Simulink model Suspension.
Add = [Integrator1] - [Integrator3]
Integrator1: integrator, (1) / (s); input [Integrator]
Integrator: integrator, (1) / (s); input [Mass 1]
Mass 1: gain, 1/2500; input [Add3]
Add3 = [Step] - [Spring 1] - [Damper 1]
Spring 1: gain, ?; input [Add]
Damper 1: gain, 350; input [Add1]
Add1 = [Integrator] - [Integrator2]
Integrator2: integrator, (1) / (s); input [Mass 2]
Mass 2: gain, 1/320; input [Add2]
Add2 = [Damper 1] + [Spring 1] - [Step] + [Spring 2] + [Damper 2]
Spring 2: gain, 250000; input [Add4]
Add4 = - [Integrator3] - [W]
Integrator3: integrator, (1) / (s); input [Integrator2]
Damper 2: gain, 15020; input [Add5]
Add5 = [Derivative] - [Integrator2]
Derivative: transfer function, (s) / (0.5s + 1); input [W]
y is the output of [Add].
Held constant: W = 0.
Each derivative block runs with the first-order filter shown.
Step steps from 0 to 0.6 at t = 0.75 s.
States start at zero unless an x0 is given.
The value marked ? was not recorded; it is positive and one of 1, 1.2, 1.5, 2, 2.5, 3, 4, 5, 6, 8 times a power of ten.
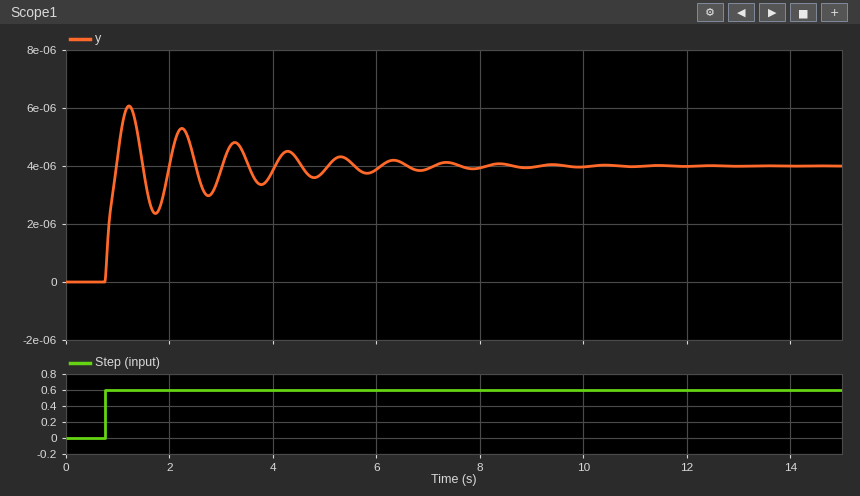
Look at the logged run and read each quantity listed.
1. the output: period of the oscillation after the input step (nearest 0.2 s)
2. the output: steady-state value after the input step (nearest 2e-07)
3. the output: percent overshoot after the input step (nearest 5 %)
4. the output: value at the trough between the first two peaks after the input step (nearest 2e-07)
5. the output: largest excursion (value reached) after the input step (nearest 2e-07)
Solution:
1.0 s
0.0000040
50 %
0.0000024
0.0000060
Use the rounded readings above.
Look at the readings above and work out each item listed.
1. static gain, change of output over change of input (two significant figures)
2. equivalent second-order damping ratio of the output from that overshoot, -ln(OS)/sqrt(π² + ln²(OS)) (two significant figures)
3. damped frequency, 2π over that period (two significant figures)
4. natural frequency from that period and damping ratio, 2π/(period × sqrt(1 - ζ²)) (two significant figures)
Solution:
0.0000067
0.22
6.3 rad/s
6.4 rad/s
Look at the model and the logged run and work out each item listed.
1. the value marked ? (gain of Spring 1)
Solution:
150000
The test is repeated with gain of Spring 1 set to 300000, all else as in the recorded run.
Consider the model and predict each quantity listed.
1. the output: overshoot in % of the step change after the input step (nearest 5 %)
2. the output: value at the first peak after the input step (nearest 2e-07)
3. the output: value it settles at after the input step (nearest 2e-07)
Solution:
35 %
0.0000026
0.0000020
